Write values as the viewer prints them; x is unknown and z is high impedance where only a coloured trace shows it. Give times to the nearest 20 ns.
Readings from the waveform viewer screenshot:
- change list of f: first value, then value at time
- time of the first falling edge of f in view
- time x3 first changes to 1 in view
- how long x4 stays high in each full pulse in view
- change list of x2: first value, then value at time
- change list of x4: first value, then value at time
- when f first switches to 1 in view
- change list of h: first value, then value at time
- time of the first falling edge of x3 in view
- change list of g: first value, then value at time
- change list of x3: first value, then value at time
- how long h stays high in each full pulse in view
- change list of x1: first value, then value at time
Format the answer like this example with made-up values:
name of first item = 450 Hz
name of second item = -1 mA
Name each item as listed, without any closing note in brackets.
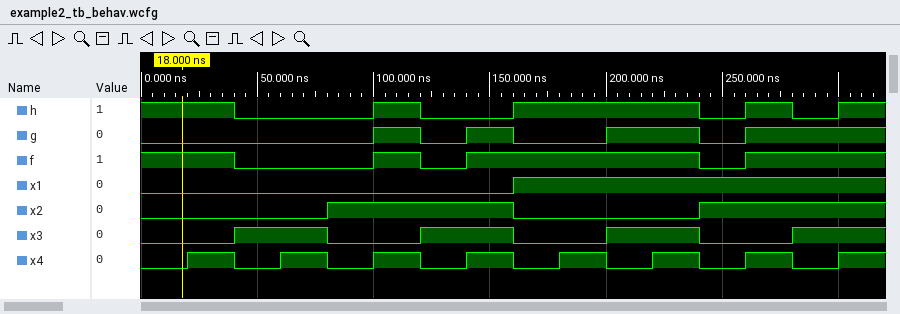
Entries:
change list of f: first value, then value at time = 1, 0 at 40 ns, 1 at 100 ns, 0 at 120 ns, 1 at 140 ns, 0 at 240 ns, 1 at 260 ns
time of the first falling edge of f in view = 40 ns
time x3 first changes to 1 in view = 40 ns
how long x4 stays high in each full pulse in view = 20 ns, 20 ns, 20 ns, 20 ns, 20 ns, 20 ns, 20 ns
change list of x2: first value, then value at time = 0, 1 at 80 ns, 0 at 160 ns, 1 at 240 ns
change list of x4: first value, then value at time = 0, 1 at 20 ns, 0 at 40 ns, 1 at 60 ns, 0 at 80 ns, 1 at 100 ns, 0 at 120 ns, 1 at 140 ns, 0 at 160 ns, 1 at 180 ns, 0 at 200 ns, 1 at 220 ns, 0 at 240 ns, 1 at 260 ns, 0 at 280 ns, 1 at 300 ns
when f first switches to 1 in view = 100 ns
change list of h: first value, then value at time = 1, 0 at 40 ns, 1 at 100 ns, 0 at 120 ns, 1 at 160 ns, 0 at 240 ns, 1 at 260 ns, 0 at 280 ns, 1 at 300 ns
time of the first falling edge of x3 in view = 80 ns
change list of g: first value, then value at time = 0, 1 at 100 ns, 0 at 120 ns, 1 at 140 ns, 0 at 160 ns, 1 at 200 ns, 0 at 240 ns, 1 at 260 ns
change list of x3: first value, then value at time = 0, 1 at 40 ns, 0 at 80 ns, 1 at 120 ns, 0 at 160 ns, 1 at 200 ns, 0 at 240 ns, 1 at 280 ns
how long h stays high in each full pulse in view = 20 ns, 80 ns, 20 ns
change list of x1: first value, then value at time = 0, 1 at 160 ns
